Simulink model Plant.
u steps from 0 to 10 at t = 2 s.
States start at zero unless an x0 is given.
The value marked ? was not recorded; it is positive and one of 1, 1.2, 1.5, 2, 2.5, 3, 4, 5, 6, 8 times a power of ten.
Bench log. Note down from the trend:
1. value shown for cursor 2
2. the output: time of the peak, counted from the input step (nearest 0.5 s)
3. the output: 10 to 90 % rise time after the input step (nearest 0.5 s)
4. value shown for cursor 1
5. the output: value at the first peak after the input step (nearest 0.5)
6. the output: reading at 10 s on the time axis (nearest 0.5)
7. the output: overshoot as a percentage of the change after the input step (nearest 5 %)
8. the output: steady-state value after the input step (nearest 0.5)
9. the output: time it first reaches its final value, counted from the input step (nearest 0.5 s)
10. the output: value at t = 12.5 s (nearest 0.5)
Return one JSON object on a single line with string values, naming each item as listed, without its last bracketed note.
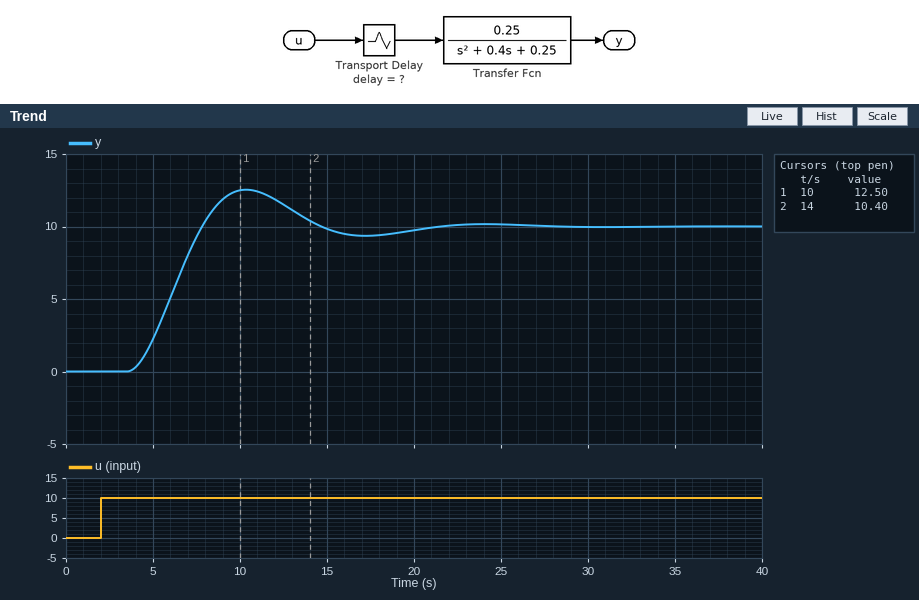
{"value shown for cursor 2": "10.40", "the output: time of the peak, counted from the input step": "8.5 s", "the output: 10 to 90 % rise time after the input step": "3.0 s", "value shown for cursor 1": "12.50", "the output: value at the first peak after the input step": "12.5", "the output: reading at 10 s on the time axis": "12.5", "the output: overshoot as a percentage of the change after the input step": "25 %", "the output: steady-state value after the input step": "10.0", "the output: time it first reaches its final value, counted from the input step": "6.0 s", "the output: value at t = 12.5 s": "11.5"}
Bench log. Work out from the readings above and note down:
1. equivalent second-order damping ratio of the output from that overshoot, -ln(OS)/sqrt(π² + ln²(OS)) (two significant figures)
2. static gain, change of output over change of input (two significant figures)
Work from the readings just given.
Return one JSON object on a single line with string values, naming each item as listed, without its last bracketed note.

{"equivalent second-order damping ratio of the output from that overshoot, -ln(OS)/sqrt(π² + ln²(OS))": "0.40", "static gain, change of output over change of input": "1.0"}
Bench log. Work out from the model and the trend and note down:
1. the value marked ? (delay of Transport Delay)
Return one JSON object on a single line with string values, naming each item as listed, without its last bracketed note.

{"the value marked ?": "1.5"}
